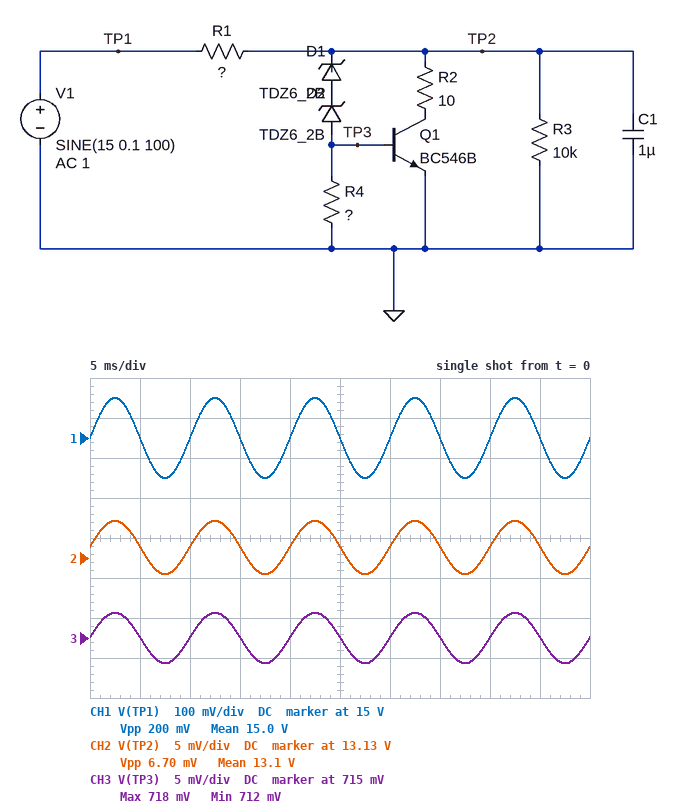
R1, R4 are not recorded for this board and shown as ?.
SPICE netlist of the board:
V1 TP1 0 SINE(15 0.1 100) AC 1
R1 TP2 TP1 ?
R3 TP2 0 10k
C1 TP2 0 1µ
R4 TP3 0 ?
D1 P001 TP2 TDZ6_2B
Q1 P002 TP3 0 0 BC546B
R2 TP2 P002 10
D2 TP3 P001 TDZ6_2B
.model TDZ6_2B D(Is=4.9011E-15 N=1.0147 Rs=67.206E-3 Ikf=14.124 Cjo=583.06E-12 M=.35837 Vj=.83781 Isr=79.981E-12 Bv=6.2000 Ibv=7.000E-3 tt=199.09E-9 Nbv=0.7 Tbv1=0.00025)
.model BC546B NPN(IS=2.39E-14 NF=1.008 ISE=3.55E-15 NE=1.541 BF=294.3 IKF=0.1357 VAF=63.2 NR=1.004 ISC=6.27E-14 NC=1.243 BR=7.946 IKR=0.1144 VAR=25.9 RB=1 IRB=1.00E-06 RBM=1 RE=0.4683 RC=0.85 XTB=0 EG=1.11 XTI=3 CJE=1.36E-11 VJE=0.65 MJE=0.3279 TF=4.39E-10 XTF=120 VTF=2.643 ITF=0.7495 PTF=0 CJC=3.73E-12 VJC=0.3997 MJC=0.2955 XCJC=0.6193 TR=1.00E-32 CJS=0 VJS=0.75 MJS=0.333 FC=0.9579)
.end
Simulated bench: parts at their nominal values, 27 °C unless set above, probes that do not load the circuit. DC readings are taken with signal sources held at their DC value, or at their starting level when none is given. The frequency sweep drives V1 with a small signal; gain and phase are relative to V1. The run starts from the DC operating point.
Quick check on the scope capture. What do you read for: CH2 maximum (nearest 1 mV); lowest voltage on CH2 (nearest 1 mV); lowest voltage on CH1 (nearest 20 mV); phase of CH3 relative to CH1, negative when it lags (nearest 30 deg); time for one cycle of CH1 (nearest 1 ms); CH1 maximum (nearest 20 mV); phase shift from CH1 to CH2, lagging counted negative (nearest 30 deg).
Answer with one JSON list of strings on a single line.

["13.135 V", "13.128 V", "14.90 V", "0 deg", "10 ms", "15.10 V", "0 deg"]
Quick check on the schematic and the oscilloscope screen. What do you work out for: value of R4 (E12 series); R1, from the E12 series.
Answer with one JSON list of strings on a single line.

["68 Ω", "68 Ω"]
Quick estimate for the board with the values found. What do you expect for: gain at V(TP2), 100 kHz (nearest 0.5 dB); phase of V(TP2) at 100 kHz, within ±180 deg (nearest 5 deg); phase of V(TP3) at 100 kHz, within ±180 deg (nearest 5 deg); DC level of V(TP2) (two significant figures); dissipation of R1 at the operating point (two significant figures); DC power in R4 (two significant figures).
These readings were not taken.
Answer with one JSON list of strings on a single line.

["-34.5 dB", "-55 deg", "-55 deg", "13 V", "51 mW", "7.5 mW"]
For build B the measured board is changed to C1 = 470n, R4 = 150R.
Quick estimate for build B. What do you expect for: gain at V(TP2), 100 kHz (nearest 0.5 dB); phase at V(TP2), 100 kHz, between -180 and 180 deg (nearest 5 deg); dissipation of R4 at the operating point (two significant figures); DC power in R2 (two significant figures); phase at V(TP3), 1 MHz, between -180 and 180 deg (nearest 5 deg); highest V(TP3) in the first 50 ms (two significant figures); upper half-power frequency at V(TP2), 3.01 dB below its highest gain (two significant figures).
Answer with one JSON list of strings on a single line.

["-32.5 dB", "-30 deg", "3.5 mW", "4.6 mW", "-80 deg", "730 mV", "180 kHz"]
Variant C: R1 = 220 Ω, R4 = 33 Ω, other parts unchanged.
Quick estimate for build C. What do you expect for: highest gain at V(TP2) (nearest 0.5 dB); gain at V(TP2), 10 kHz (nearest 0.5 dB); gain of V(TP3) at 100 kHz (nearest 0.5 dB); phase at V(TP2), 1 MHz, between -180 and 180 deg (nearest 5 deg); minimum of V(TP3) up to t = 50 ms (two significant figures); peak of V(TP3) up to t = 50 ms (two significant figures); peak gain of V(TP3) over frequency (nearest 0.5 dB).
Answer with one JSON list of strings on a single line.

["-17.0 dB", "-24.0 dB", "-44.0 dB", "-90 deg", "290 mV", "310 mV", "-18.0 dB"]
